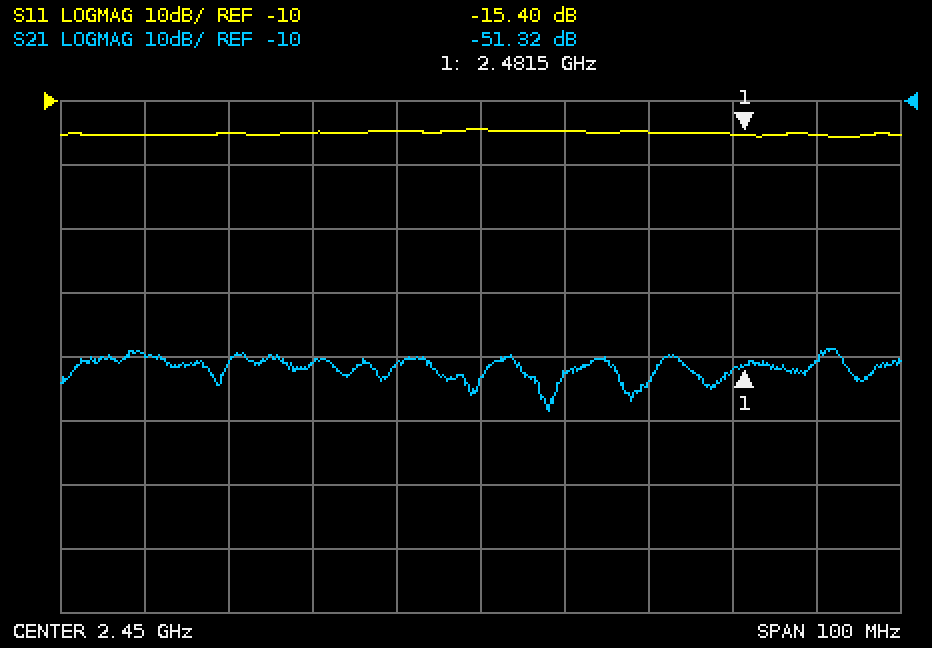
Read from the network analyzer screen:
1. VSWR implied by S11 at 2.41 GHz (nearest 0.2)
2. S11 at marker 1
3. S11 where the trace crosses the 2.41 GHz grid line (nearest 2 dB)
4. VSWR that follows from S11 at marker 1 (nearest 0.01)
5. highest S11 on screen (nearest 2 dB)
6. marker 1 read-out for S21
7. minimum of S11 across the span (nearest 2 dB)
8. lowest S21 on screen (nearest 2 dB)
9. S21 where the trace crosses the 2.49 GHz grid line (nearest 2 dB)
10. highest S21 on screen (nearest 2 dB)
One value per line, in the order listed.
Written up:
1.4
-15.40 dB
-16 dB
1.41
-14 dB
-51.32 dB
-16 dB
-58 dB
-50 dB
-48 dB
